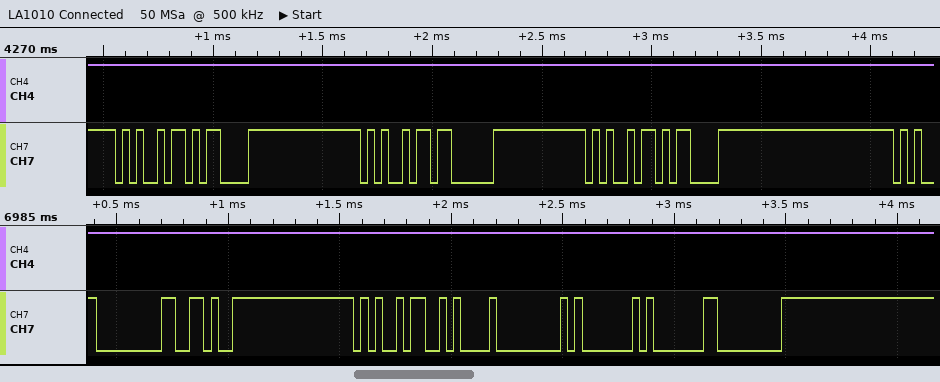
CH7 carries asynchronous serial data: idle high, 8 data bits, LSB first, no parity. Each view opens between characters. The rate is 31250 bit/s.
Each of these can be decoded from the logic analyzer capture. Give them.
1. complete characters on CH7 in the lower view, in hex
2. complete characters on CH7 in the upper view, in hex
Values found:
00, 96, A5, 0A, 00, 01, 01, 00
A5, 0D, A5, 03, A5, 0D
